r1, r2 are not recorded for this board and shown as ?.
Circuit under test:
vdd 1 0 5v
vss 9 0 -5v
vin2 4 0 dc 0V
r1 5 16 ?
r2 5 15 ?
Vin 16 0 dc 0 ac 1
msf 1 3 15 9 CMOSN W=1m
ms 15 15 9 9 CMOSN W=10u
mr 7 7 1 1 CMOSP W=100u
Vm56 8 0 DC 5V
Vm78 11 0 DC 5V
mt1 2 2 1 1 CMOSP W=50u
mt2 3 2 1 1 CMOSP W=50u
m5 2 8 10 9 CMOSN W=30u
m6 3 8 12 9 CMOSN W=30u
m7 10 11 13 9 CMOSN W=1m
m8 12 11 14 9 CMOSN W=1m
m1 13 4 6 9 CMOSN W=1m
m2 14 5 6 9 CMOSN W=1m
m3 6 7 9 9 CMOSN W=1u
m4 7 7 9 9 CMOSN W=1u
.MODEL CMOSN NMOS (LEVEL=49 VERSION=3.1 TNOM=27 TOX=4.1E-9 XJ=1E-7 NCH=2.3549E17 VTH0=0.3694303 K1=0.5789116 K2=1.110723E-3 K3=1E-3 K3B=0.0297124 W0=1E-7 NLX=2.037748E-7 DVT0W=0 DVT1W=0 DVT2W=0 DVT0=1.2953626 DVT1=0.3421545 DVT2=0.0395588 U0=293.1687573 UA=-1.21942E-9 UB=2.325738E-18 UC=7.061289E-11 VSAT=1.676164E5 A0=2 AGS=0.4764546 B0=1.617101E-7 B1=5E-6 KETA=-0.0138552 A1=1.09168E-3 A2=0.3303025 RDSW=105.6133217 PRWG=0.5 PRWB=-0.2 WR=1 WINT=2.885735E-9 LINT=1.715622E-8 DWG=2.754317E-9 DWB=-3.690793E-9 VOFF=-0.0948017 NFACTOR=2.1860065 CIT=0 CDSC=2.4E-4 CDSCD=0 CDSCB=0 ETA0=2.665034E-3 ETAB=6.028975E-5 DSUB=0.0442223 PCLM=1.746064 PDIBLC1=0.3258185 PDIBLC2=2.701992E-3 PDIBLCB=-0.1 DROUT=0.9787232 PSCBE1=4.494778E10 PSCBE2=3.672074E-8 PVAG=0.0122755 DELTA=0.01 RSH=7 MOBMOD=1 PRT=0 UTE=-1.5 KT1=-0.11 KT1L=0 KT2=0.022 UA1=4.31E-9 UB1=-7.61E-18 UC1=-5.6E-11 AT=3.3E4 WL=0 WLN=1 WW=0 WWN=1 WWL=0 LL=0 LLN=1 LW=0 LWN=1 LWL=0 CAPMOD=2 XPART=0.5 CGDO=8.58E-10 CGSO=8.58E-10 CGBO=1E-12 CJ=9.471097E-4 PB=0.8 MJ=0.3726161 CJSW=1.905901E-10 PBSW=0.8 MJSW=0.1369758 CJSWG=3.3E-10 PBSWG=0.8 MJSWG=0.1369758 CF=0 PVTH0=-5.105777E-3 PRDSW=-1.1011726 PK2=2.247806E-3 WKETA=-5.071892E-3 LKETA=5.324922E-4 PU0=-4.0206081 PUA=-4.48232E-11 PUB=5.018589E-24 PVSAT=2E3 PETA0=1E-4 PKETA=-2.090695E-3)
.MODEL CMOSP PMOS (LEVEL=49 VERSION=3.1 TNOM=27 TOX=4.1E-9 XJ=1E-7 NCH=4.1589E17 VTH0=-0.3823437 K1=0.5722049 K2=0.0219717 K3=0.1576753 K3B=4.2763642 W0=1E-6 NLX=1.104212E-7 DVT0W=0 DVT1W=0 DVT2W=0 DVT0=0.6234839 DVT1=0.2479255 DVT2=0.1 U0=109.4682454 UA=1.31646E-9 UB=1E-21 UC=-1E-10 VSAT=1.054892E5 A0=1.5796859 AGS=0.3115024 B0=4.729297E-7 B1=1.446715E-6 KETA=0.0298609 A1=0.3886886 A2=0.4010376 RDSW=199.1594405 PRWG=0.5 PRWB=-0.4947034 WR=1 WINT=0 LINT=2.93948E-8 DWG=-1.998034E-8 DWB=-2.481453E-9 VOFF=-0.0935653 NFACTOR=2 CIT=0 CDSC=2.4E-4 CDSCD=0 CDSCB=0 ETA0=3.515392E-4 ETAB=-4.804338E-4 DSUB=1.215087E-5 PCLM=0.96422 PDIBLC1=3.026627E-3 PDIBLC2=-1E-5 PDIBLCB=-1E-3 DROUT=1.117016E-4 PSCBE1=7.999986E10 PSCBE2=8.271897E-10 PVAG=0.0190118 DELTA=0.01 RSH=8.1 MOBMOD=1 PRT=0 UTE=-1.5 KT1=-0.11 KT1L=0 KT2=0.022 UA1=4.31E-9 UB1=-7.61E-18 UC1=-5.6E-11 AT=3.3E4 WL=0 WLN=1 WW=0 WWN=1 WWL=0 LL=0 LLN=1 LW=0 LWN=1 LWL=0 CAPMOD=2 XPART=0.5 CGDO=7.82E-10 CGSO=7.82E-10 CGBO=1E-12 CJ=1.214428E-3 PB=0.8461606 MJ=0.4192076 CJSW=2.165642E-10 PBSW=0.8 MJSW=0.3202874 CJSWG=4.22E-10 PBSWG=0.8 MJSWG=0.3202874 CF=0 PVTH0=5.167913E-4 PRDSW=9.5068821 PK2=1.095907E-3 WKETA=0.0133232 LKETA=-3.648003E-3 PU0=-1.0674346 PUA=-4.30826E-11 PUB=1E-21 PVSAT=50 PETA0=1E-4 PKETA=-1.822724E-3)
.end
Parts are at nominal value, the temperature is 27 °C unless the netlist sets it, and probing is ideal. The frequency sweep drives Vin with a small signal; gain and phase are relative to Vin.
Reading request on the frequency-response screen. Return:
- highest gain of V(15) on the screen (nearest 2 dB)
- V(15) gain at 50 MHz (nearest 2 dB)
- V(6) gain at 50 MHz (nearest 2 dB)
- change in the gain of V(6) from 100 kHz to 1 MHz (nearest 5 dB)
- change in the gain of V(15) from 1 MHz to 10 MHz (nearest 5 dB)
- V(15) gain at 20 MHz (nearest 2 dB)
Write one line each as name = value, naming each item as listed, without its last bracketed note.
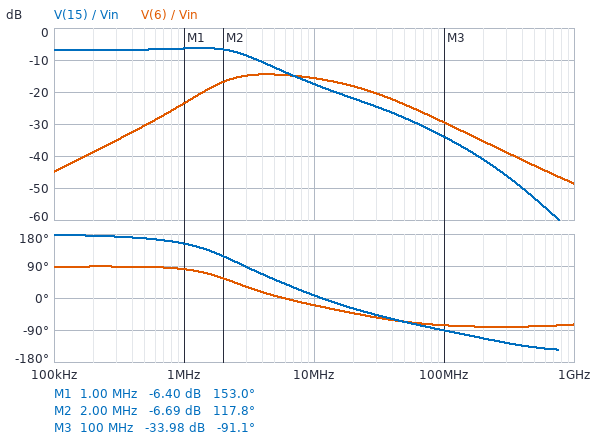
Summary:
highest gain of V(15) on the screen = -6 dB
V(15) gain at 50 MHz = -28 dB
V(6) gain at 50 MHz = -24 dB
change in the gain of V(6) from 100 kHz to 1 MHz = 20 dB
change in the gain of V(15) from 1 MHz to 10 MHz = -10 dB
V(15) gain at 20 MHz = -22 dB
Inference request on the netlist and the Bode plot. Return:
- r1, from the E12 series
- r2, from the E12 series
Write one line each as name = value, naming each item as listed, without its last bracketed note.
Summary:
r1, from the E12 series = 1.5 kΩ
r2, from the E12 series = 680 Ω
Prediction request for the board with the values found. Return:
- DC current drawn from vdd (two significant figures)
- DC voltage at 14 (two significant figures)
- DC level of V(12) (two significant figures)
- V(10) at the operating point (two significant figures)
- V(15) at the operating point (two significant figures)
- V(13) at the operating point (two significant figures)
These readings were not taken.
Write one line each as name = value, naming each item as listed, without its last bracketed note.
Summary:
DC current drawn from vdd = 3.0 mA
DC voltage at 14 = 1.5 V
DC level of V(12) = 1.5 V
V(10) at the operating point = 3.1 V
V(15) at the operating point = 6.9 mV
V(13) at the operating point = 3.1 V
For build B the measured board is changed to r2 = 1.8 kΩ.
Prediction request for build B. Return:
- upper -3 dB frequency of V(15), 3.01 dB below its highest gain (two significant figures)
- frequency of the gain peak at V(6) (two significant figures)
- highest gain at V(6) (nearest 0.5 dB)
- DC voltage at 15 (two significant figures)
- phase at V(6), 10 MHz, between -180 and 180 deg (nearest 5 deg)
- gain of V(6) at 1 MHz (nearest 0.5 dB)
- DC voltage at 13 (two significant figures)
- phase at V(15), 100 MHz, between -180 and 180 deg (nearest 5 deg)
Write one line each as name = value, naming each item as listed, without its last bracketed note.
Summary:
upper -3 dB frequency of V(15), 3.01 dB below its highest gain = 2.2 MHz
frequency of the gain peak at V(6) = 2.9 MHz
highest gain at V(6) = -10.5 dB
DC voltage at 15 = 10 mV
phase at V(6), 10 MHz, between -180 and 180 deg = -35 deg
gain of V(6) at 1 MHz = -16.0 dB
DC voltage at 13 = 3.1 V
phase at V(15), 100 MHz, between -180 and 180 deg = -100 deg
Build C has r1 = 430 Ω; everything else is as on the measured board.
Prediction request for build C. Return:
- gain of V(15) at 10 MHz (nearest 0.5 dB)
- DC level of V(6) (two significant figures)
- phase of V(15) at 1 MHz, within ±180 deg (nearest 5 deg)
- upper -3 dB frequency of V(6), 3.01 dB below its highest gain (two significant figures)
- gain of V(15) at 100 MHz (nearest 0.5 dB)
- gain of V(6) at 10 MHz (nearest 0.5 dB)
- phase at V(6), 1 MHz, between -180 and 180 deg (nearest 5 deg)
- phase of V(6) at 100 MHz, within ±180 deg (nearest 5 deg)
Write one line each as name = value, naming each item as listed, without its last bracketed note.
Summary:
gain of V(15) at 10 MHz = -12.0 dB
DC level of V(6) = -1.1 V
phase of V(15) at 1 MHz, within ±180 deg = 135 deg
upper -3 dB frequency of V(6), 3.01 dB below its highest gain = 34 MHz
gain of V(15) at 100 MHz = -23.5 dB
gain of V(6) at 10 MHz = -10.5 dB
phase at V(6), 1 MHz, between -180 and 180 deg = 60 deg
phase of V(6) at 100 MHz, within ±180 deg = -65 deg
